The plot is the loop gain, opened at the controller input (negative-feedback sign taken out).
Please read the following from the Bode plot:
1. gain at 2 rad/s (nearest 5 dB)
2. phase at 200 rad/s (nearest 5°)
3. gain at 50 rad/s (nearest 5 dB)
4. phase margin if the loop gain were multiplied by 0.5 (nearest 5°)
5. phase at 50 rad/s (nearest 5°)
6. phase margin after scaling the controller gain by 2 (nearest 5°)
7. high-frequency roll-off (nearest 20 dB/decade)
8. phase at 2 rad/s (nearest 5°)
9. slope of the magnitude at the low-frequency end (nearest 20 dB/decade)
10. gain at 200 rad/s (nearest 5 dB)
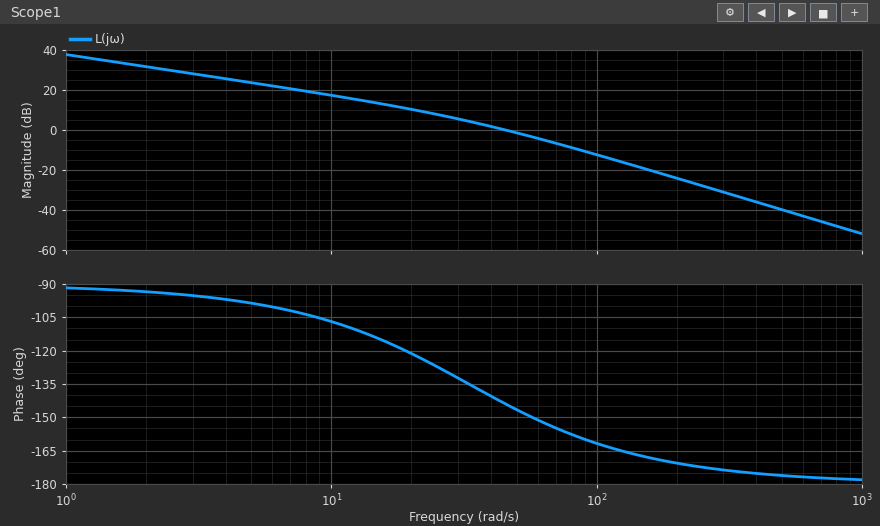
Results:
30 dB
-170°
0 dB
50°
-145°
25°
-40 dB/decade
-95°
-20 dB/decade
-25 dB
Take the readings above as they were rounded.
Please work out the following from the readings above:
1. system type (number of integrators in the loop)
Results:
1
